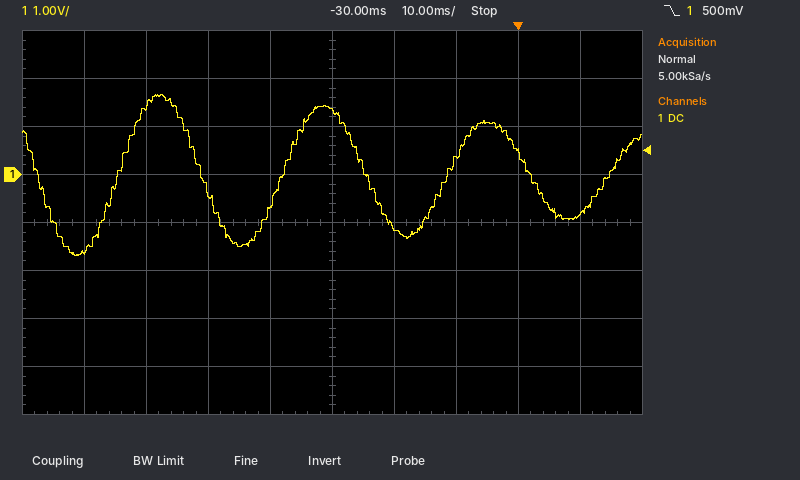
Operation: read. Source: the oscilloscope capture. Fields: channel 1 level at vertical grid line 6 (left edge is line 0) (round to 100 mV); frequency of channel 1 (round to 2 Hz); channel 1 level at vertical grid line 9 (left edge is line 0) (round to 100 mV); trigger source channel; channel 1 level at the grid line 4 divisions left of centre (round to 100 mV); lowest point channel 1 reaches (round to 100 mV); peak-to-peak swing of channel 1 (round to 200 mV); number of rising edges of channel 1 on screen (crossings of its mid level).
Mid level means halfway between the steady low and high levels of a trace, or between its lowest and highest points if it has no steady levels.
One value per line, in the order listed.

-1.1 V
38 Hz
-800 mV
channel 1
-1.6 V
-1.7 V
3.4 V
4
